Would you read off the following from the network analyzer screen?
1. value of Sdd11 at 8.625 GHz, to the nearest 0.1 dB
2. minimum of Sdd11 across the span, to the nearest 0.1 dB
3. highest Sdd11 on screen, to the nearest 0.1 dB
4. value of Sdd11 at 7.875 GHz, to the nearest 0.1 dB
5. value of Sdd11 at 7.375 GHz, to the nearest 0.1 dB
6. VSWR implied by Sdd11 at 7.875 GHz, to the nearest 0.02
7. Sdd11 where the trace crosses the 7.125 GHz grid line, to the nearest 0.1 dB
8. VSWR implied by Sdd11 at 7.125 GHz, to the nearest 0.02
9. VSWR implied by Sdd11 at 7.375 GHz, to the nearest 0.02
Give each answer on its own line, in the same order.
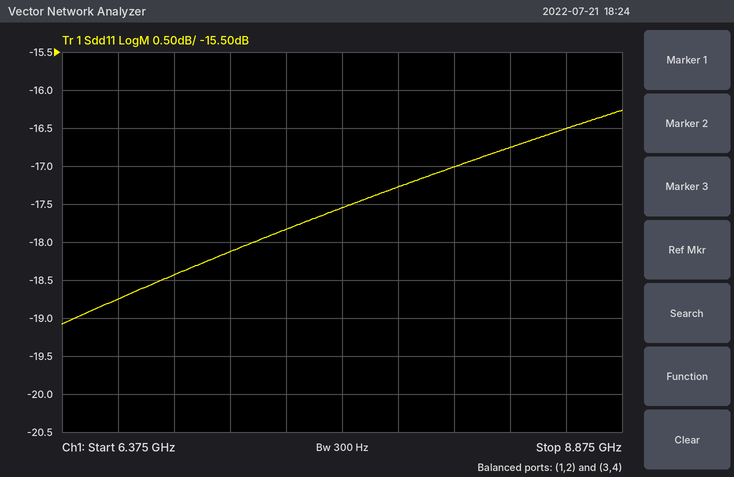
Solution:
-16.5 dB
-19.1 dB
-16.3 dB
-17.3 dB
-17.8 dB
1.32
-18.1 dB
1.28
1.30
